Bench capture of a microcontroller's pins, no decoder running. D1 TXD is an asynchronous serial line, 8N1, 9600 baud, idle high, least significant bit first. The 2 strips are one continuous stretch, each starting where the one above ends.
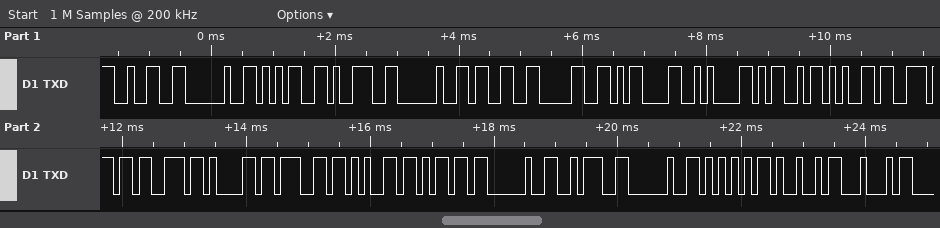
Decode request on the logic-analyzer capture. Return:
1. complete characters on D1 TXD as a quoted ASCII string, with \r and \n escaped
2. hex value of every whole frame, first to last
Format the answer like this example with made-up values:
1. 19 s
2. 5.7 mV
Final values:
1. "2 59 30\r\nMensagem : UID"
2. 32 20 35 39 20 33 30 0D 0A 4D 65 6E 73 61 67 65 6D 20 3A 20 55 49 44
